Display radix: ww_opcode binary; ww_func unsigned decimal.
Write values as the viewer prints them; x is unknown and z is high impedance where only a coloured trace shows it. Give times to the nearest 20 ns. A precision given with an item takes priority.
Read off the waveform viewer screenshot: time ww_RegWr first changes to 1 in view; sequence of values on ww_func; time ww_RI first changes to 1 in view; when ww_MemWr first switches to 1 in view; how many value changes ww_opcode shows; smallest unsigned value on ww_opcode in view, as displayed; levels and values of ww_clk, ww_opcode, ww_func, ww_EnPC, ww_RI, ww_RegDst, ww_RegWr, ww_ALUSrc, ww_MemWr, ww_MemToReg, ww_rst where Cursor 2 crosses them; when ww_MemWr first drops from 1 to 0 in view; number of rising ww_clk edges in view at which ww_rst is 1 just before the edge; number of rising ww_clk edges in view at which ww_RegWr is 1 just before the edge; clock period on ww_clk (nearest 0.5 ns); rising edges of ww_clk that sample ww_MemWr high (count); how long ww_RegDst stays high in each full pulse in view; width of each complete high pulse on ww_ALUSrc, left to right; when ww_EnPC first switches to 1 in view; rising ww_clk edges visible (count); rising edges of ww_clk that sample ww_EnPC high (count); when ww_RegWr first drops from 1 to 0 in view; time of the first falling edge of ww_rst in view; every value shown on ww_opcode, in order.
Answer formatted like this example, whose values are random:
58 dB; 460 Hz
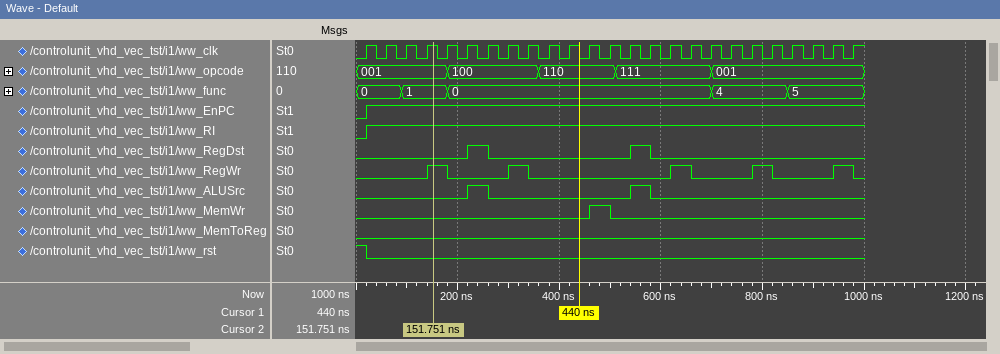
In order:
140 ns; 0, 1, 0, 4, 5; 20 ns; 460 ns; 4; 001; ww_clk=1, ww_opcode=001, ww_func=1, ww_EnPC=1, ww_RI=1, ww_RegDst=0, ww_RegWr=1, ww_ALUSrc=0, ww_MemWr=0, ww_MemToReg=0, ww_rst=0; 500 ns; 1; 5; 40 ns; 1; 40 ns, 40 ns; 40 ns, 40 ns; 20 ns; 25; 24; 180 ns; 20 ns; 001, 100, 110, 111, 001
